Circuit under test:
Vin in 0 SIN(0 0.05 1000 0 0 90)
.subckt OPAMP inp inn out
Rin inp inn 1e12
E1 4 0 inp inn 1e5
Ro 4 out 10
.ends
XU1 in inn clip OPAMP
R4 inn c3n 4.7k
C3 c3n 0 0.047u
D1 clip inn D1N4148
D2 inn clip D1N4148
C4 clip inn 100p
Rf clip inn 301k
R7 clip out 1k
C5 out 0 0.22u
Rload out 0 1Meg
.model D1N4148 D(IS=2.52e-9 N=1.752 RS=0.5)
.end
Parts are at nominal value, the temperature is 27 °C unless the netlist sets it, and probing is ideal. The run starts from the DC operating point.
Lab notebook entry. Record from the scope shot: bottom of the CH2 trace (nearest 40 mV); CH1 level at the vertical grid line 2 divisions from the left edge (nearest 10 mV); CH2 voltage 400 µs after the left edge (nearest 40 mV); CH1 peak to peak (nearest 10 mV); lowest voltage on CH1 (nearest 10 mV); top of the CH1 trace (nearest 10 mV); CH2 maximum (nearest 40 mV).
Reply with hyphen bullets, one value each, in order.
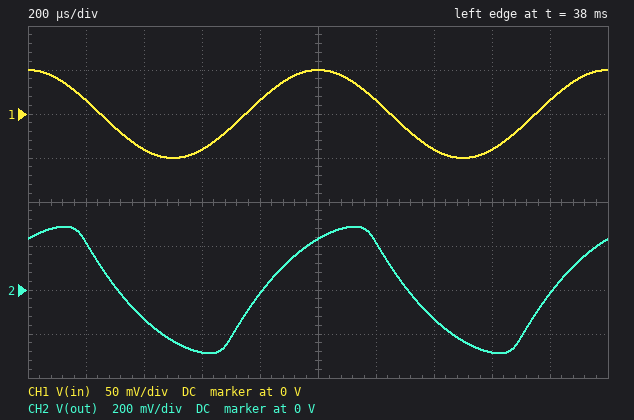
- -280 mV
- -40 mV
- -120 mV
- 100 mV
- -50 mV
- 50 mV
- 280 mV
